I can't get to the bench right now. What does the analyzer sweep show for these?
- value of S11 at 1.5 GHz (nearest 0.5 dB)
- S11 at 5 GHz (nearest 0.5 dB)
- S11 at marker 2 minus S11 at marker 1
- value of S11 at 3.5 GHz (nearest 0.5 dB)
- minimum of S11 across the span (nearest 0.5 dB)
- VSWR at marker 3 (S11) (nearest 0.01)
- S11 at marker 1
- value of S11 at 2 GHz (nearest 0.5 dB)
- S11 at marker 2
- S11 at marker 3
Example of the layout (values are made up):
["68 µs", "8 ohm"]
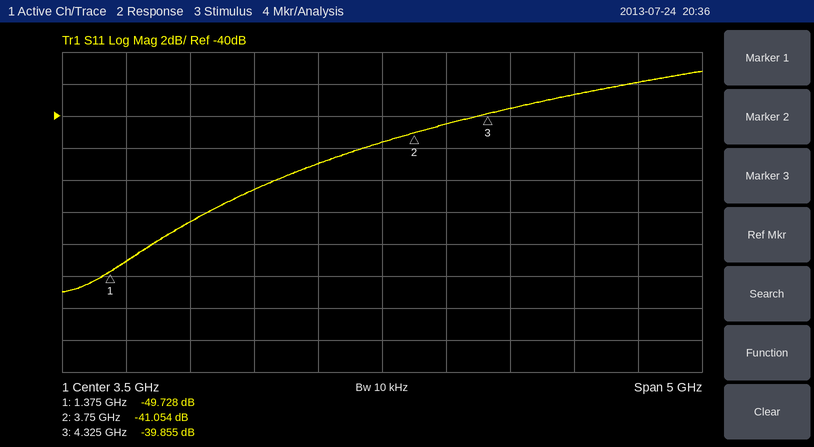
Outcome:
["-49.0 dB", "-38.5 dB", "8.674 dB", "-41.5 dB", "-51.0 dB", "1.02", "-49.728 dB", "-46.5 dB", "-41.054 dB", "-39.855 dB"]
